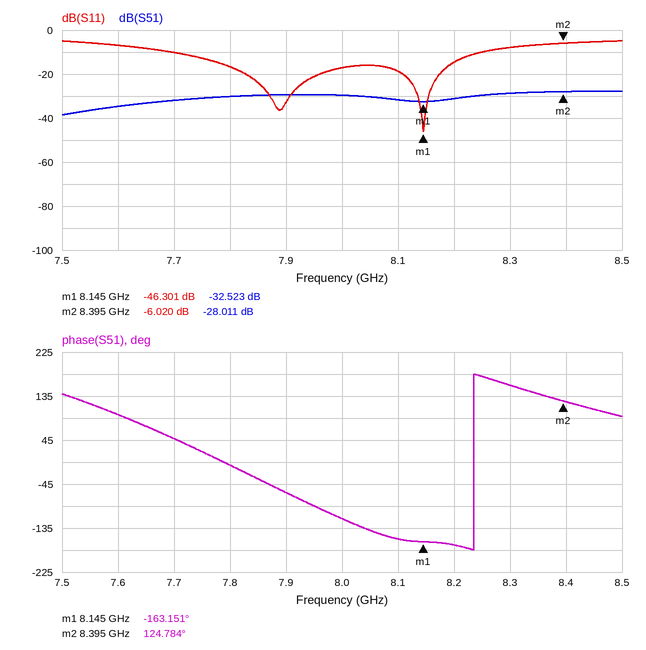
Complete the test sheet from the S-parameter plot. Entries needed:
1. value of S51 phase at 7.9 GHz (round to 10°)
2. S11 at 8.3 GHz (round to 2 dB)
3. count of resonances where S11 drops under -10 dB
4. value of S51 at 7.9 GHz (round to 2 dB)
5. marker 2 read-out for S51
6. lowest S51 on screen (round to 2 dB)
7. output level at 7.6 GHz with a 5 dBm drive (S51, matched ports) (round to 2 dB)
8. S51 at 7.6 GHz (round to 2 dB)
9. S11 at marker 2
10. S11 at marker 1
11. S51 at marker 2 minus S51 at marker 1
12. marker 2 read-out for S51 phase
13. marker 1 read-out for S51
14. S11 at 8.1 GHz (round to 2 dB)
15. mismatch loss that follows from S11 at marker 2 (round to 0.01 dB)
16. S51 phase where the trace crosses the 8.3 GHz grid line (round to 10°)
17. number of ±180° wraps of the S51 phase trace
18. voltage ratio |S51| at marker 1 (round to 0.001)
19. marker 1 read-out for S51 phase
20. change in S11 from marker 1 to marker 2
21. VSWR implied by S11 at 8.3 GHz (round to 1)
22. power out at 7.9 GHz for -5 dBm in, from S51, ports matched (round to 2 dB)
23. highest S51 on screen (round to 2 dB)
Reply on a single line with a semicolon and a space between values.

-60°; -8 dB; 2; -30 dB; -28.011 dB; -38 dB; -30 dBm; -34 dB; -6.020 dB; -46.301 dB; 4.512 dB; 124.784°; -32.523 dB; -18 dB; 1.25 dB; 160°; 1; 0.024; -163.151°; 40.281 dB; 2; -34 dBm; -28 dB
